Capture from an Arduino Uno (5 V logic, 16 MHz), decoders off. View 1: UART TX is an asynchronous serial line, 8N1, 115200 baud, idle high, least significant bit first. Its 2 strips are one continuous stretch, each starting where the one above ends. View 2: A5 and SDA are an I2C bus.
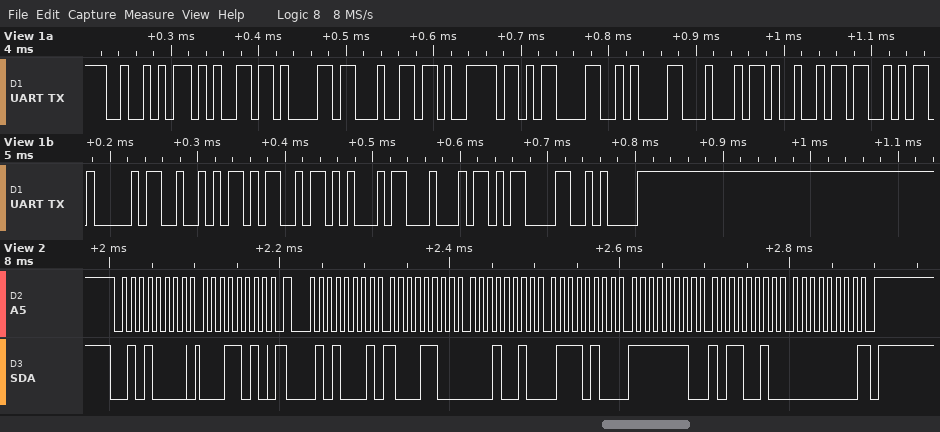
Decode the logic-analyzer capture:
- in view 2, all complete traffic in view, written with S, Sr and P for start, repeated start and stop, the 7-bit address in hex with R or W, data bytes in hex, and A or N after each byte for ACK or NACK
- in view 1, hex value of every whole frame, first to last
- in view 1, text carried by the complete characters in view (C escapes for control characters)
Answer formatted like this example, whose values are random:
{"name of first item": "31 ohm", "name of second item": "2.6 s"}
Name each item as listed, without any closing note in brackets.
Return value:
{"in view 2, all complete traffic in view, written with S, Sr and P for start, repeated start and stop, the 7-bit address in hex with R or W, data bytes in hex, and A or N after each byte for ACK or NACK": "S 28W A 1A A Sr 28R A 8C A 12 A 74 A FE A B2 A 00 N P", "in view 1, hex value of every whole frame, first to last": "52 65 61 64 79 0D 0A 44 49 53 41 52 4D 45 44 0D 0A", "in view 1, text carried by the complete characters in view": "\"Ready\\r\\nDISARMED\\r\\n\""}
